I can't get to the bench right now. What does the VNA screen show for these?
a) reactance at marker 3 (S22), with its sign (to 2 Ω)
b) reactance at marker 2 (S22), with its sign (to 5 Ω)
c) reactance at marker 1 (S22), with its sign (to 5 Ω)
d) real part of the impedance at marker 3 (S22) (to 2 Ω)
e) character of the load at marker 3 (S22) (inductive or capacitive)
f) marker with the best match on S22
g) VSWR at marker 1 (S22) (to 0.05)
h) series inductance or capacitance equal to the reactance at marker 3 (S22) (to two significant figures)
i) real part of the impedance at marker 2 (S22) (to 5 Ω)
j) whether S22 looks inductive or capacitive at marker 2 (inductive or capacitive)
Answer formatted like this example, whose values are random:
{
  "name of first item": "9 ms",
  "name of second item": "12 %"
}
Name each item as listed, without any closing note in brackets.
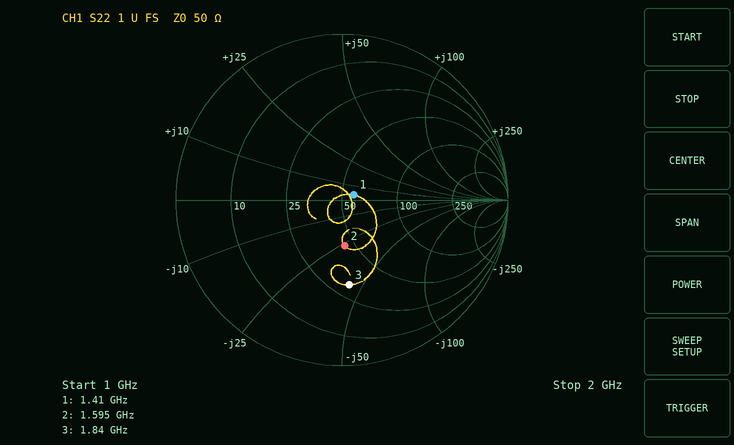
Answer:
{
  "reactance at marker 3 (S22), with its sign": "-44 Ω",
  "reactance at marker 2 (S22), with its sign": "-25 Ω",
  "reactance at marker 1 (S22), with its sign": "+5 Ω",
  "real part of the impedance at marker 3 (S22)": "32 Ω",
  "character of the load at marker 3 (S22)": "capacitive",
  "marker with the best match on S22": "marker 1",
  "VSWR at marker 1 (S22)": "1.15",
  "series inductance or capacitance equal to the reactance at marker 3 (S22)": "2.0 pF",
  "real part of the impedance at marker 2 (S22)": "45 Ω",
  "whether S22 looks inductive or capacitive at marker 2": "capacitive"
}
